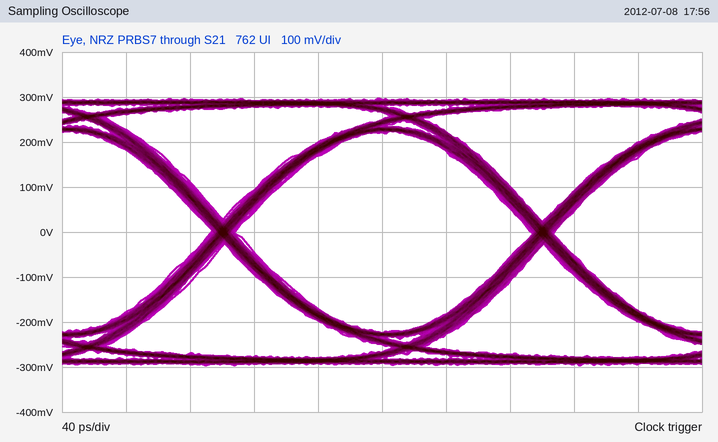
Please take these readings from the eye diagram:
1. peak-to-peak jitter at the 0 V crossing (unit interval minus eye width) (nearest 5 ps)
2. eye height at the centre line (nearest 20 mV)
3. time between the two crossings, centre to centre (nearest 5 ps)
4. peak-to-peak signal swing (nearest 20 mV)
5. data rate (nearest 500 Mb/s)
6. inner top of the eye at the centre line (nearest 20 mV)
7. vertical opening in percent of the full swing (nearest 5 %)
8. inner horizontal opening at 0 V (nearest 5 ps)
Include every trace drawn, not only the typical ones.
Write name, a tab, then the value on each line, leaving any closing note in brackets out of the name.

peak-to-peak jitter at the 0 V crossing (unit interval minus eye width)	15 ps
eye height at the centre line	440 mV
time between the two crossings, centre to centre	200 ps
peak-to-peak signal swing	600 mV
data rate	5.0 Gb/s
inner top of the eye at the centre line	220 mV
vertical opening in percent of the full swing	75 %
inner horizontal opening at 0 V	185 ps
